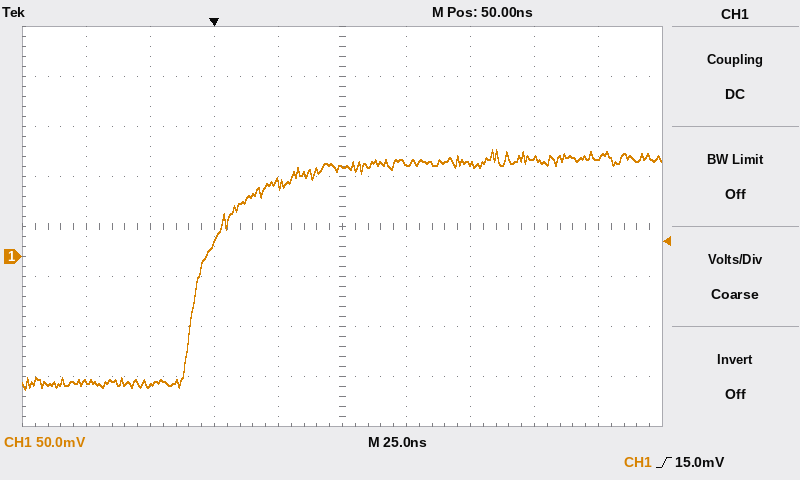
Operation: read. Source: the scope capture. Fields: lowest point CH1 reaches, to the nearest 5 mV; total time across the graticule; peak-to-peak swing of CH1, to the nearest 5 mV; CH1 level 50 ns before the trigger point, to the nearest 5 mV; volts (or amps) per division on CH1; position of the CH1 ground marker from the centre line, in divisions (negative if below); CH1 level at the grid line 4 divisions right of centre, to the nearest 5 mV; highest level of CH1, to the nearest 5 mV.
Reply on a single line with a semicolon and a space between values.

-135 mV; 250 ns; 240 mV; -125 mV; 50 mV; -0.6 div; 100 mV; 105 mV
